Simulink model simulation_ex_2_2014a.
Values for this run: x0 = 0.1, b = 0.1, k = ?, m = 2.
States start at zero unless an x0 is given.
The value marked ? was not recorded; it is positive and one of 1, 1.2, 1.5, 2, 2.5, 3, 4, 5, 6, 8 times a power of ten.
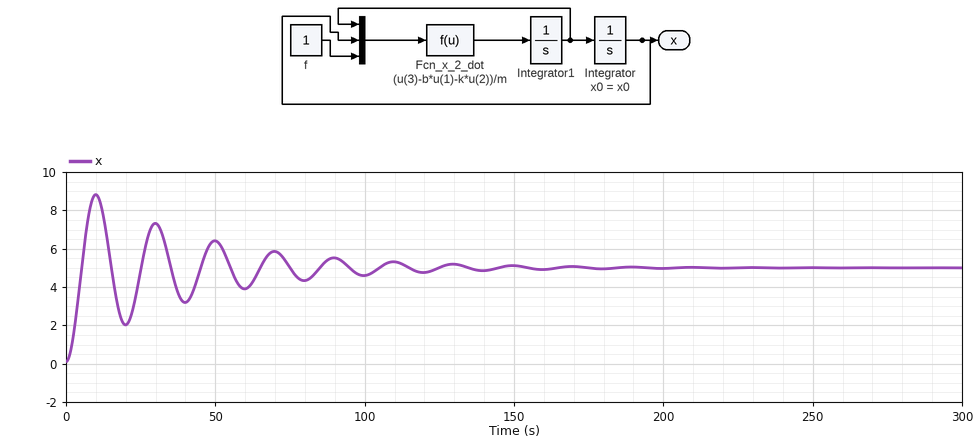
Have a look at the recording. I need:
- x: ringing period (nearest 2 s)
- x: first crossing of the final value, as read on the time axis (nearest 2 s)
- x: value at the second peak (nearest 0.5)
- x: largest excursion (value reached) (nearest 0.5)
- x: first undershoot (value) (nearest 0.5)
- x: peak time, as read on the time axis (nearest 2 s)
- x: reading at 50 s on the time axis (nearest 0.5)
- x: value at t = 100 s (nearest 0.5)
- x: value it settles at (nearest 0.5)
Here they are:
20 s
6 s
7.5
9.0
2.0
10 s
6.5
4.5
5.0
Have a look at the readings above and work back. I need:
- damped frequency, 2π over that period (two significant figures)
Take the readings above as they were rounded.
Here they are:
0.31 rad/s
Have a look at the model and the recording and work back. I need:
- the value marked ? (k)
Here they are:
0.2
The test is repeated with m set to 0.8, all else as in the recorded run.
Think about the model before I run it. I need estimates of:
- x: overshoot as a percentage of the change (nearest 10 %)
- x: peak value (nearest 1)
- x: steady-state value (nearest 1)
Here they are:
70 %
8
5
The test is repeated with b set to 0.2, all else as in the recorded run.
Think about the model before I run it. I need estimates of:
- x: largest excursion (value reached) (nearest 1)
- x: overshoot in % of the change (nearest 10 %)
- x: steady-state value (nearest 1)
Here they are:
8
60 %
5
